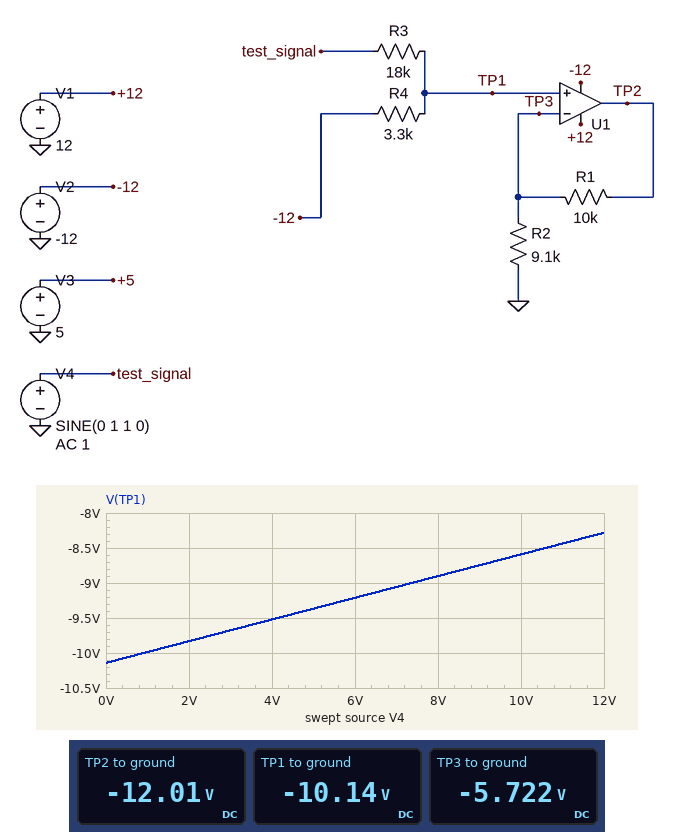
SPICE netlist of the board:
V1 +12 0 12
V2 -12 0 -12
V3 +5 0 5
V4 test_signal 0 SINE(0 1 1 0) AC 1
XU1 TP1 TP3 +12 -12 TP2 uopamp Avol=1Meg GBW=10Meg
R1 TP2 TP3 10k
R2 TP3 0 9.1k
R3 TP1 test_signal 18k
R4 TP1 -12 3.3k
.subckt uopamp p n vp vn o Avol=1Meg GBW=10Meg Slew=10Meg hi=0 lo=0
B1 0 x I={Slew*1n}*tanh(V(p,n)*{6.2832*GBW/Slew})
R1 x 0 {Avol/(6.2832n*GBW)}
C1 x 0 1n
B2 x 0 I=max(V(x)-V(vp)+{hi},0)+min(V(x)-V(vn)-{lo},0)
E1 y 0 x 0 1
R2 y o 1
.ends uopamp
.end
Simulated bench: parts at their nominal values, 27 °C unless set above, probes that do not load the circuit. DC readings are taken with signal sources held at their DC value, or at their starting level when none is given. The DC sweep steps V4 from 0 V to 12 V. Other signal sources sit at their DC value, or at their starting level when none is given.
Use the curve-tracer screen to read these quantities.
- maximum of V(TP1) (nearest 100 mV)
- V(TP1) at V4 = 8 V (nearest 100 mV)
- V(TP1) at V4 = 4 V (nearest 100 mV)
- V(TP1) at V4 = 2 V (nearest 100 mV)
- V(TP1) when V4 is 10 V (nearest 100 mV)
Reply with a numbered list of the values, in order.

1. -8.3 V
2. -8.9 V
3. -9.5 V
4. -9.8 V
5. -8.6 V
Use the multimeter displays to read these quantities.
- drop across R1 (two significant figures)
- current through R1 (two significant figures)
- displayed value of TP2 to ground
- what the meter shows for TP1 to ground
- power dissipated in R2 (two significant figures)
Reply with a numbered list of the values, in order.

1. 6.3 V
2. 630 µA
3. -12.01 V
4. -10.14 V
5. 3.6 mW
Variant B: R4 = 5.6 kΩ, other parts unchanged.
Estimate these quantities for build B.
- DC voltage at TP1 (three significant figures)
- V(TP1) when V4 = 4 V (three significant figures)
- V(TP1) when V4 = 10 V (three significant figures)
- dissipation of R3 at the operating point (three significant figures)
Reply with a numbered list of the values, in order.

1. -9.15 V
2. -8.20 V
3. -6.78 V
4. 4.65 mW
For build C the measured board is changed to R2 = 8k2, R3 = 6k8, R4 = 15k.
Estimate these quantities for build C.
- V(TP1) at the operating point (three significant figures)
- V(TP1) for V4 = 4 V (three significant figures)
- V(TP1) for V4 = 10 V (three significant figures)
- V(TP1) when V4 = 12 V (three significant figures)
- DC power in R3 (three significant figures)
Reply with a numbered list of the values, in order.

1. -3.74 V
2. -991 mV
3. 3.14 V
4. 4.51 V
5. 2.06 mW
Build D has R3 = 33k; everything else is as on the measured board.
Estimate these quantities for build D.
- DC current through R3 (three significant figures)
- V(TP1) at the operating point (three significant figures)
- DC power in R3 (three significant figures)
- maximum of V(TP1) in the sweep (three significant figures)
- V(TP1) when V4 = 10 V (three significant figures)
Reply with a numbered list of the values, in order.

1. 331 µA
2. -10.9 V
3. 3.61 mW
4. -9.82 V
5. -10.0 V
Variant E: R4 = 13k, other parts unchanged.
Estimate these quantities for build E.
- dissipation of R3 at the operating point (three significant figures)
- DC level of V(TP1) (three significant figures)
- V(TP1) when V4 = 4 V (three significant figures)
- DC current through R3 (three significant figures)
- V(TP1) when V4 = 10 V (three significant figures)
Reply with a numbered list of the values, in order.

1. 2.70 mW
2. -6.97 V
3. -5.29 V
4. 387 µA
5. -2.77 V
